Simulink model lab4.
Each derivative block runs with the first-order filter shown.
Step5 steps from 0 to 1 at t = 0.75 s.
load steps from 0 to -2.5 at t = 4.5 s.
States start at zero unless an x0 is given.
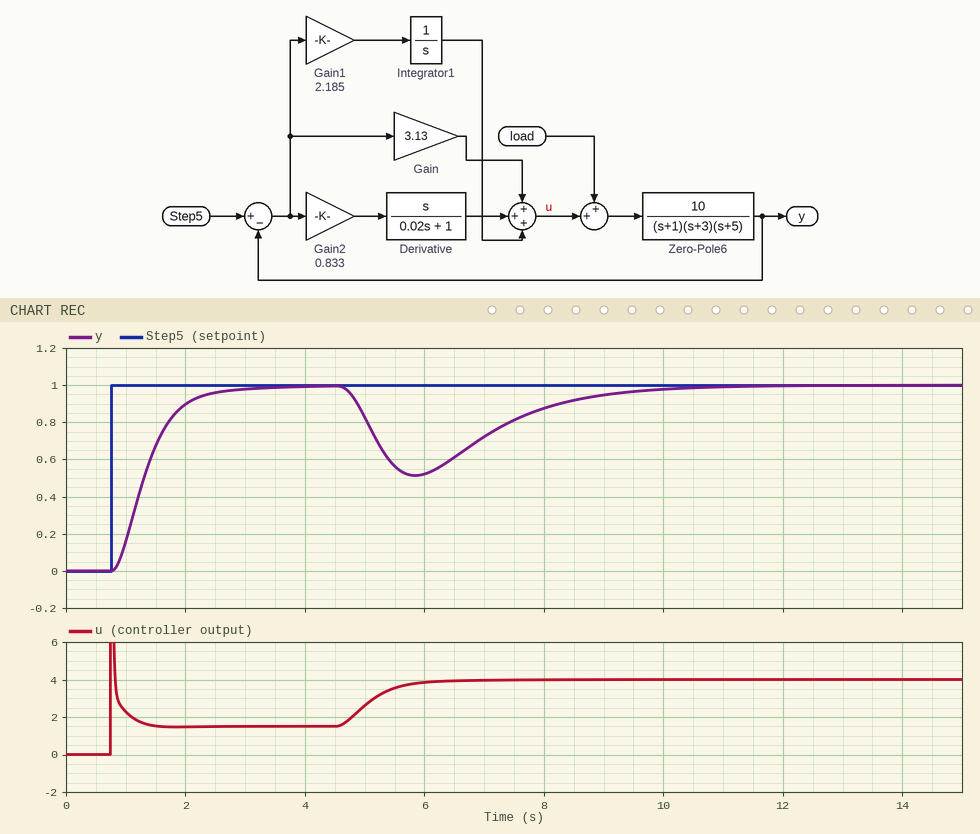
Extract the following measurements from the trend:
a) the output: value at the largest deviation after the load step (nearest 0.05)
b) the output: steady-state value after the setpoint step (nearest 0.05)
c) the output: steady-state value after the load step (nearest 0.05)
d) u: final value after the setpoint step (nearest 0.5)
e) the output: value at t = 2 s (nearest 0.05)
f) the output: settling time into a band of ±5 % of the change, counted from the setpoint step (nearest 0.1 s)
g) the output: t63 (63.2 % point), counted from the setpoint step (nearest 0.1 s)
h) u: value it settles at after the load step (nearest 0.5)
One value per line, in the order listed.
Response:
0.50
1.00
1.00
1.5
0.90
1.6 s
0.7 s
4.0
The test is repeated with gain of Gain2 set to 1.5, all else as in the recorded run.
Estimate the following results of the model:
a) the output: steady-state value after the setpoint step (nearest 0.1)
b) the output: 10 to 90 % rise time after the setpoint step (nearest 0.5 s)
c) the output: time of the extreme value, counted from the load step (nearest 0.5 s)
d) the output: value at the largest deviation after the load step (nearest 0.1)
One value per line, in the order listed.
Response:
1.0
1.5 s
1.5 s
0.6
